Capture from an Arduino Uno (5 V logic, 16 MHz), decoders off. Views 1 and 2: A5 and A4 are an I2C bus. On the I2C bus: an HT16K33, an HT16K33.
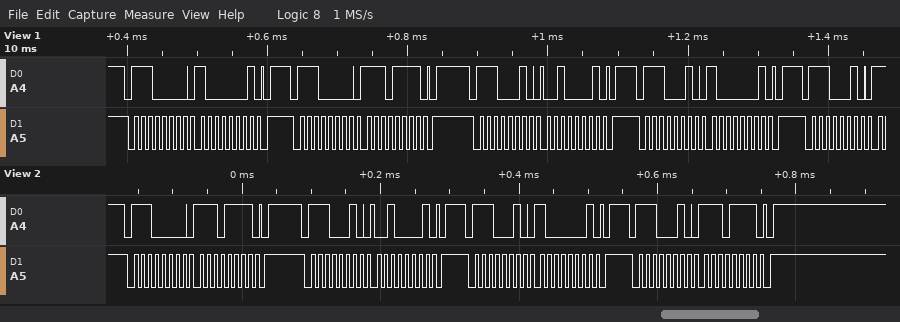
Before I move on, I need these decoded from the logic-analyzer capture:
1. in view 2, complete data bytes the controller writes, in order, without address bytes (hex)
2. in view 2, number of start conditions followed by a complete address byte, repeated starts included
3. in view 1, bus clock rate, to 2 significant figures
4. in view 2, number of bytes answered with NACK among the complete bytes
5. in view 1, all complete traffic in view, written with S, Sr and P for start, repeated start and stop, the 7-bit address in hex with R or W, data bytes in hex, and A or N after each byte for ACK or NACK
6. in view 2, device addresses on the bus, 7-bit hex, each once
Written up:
EF 21 81 EF
4
100 kHz
0
S 70W A 81 A P S 70W A EF A P S 71W A 21 A P S 71W A 81 A P S 71W A
0x70 0x71
